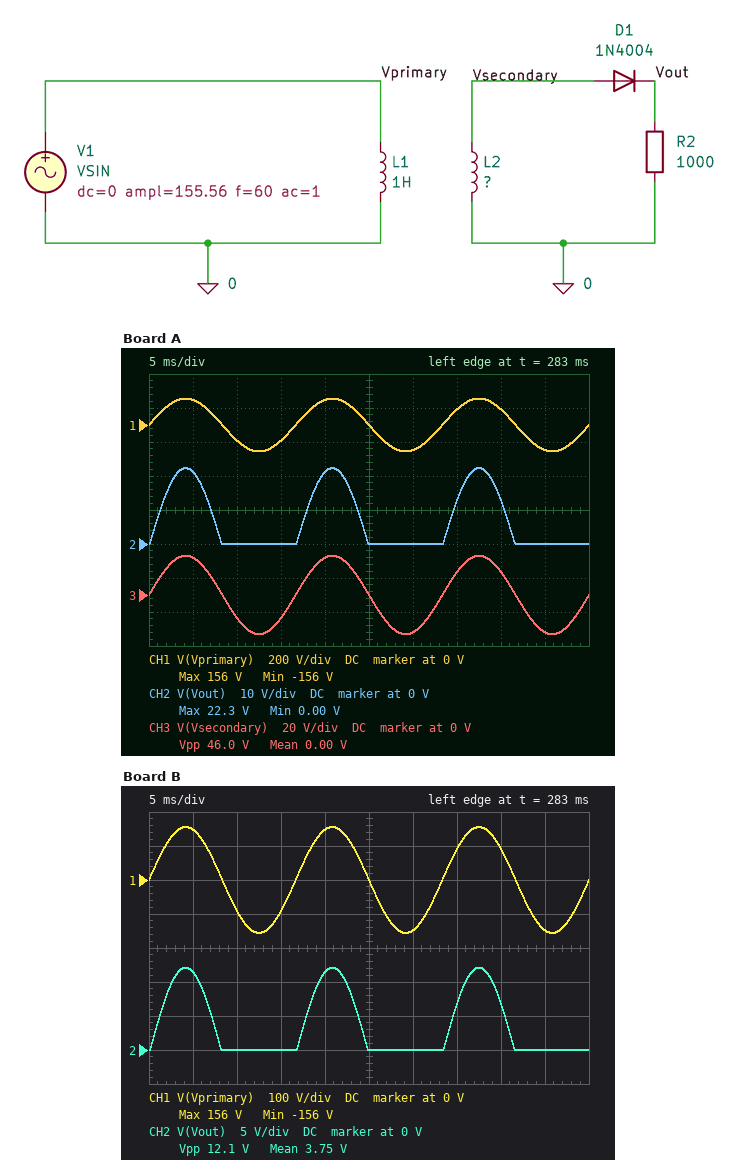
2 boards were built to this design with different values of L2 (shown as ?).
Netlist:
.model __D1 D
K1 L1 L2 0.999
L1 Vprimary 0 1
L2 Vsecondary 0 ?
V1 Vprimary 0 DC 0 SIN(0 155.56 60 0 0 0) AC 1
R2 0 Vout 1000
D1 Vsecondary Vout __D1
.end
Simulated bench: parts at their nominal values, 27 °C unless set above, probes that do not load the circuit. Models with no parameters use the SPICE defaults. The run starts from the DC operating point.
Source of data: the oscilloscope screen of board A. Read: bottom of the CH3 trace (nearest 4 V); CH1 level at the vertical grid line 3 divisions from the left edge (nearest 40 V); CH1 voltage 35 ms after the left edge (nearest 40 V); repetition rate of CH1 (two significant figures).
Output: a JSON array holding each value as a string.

["-24 V", "-80 V", "80 V", "60 Hz"]
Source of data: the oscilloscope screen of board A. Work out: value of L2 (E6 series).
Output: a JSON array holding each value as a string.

["22 mH"]
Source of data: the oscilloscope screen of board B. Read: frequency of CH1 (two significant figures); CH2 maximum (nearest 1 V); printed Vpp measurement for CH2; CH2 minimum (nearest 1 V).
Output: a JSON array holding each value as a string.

["60 Hz", "12 V", "12.1 V", "0 V"]
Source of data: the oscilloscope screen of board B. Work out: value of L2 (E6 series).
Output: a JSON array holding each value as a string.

["6.8 mH"]
